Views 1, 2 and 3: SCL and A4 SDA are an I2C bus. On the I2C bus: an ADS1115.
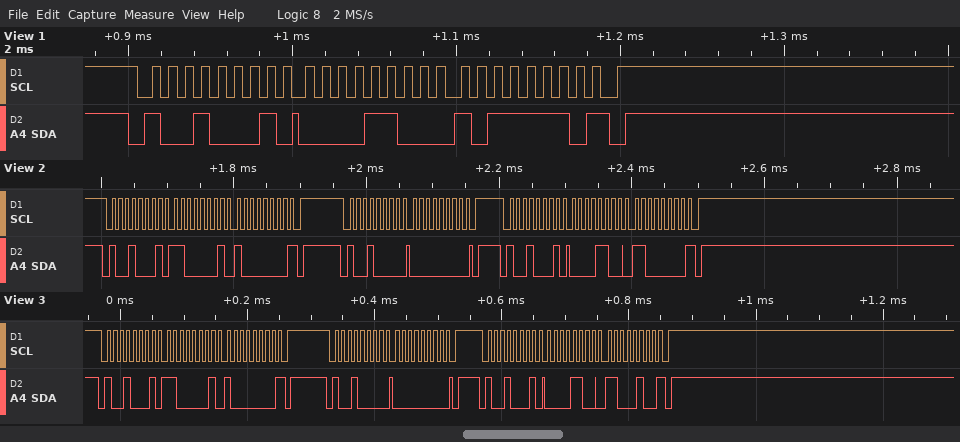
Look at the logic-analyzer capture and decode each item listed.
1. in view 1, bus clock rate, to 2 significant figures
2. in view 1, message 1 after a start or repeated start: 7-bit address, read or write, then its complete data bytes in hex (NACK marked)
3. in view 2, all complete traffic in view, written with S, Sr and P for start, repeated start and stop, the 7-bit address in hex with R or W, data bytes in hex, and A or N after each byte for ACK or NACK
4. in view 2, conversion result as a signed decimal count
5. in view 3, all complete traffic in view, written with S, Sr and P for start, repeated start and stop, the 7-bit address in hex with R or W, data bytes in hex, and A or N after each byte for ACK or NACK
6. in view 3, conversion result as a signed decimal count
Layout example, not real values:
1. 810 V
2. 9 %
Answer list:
1. 100 kHz
2. 0x48 read: 0C BE NACK
3. S 48R A C1 A 80 N P S 48W A 00 A P S 48R A 0C A C0 N P
4. 3264
5. S 48R A C1 A 80 N P S 48W A 00 A P S 48R A 0C A C4 N P
6. 3268
